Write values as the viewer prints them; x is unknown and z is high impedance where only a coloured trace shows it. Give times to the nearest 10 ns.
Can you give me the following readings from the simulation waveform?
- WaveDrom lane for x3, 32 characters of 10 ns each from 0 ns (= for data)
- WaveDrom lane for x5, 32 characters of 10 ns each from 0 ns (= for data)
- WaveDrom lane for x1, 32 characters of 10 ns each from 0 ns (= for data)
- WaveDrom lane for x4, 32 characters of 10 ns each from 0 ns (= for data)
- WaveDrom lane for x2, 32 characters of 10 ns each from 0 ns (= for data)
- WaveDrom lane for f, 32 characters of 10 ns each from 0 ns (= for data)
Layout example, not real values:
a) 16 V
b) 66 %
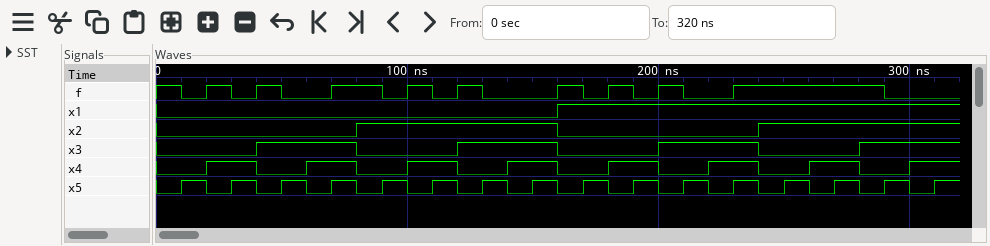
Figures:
a) {name: 'x3', wave: '0...1...0...1...0...1...0...1...'}
b) {name: 'x5', wave: '01010101010101010101010101010101'}
c) {name: 'x1', wave: '0...............1...............'}
d) {name: 'x4', wave: '0.1.0.1.0.1.0.1.0.1.0.1.0.1.0.1.'}
e) {name: 'x2', wave: '0.......1.......0.......1.......'}
f) {name: 'f', wave: '101010.1.01010..101010.1.....0..'}
